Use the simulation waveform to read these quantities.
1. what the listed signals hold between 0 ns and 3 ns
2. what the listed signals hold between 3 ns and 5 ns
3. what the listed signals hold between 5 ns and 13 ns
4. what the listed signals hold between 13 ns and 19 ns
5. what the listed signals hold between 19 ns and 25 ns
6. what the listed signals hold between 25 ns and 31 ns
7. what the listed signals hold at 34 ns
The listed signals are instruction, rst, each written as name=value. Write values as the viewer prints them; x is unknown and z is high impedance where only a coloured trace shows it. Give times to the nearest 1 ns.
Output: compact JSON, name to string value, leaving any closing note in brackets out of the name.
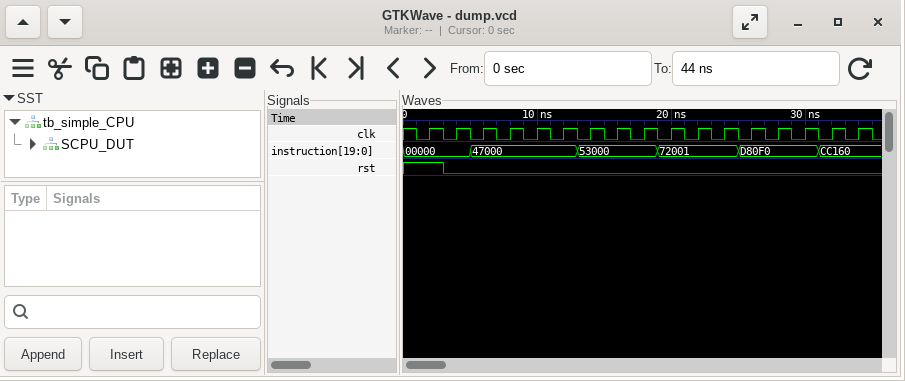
{"what the listed signals hold between 0 ns and 3 ns": "instruction=00000, rst=1", "what the listed signals hold between 3 ns and 5 ns": "instruction=00000, rst=0", "what the listed signals hold between 5 ns and 13 ns": "instruction=47000, rst=0", "what the listed signals hold between 13 ns and 19 ns": "instruction=53000, rst=0", "what the listed signals hold between 19 ns and 25 ns": "instruction=72001, rst=0", "what the listed signals hold between 25 ns and 31 ns": "instruction=D80F0, rst=0", "what the listed signals hold at 34 ns": "instruction=CC160, rst=0"}
